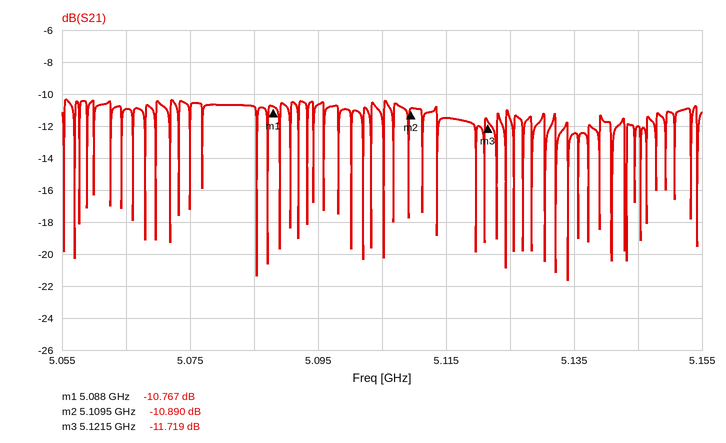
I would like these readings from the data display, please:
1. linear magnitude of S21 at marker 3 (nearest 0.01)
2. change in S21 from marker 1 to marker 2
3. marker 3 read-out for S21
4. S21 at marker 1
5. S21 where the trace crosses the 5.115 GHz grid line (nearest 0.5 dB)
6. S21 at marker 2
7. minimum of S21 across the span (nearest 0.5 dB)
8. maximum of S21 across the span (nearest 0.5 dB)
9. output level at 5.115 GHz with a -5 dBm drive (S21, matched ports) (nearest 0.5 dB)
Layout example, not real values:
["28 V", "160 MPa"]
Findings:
["0.26", "-0.123 dB", "-11.719 dB", "-10.767 dB", "-11.5 dB", "-10.890 dB", "-21.5 dB", "-10.5 dB", "-16.5 dBm"]
